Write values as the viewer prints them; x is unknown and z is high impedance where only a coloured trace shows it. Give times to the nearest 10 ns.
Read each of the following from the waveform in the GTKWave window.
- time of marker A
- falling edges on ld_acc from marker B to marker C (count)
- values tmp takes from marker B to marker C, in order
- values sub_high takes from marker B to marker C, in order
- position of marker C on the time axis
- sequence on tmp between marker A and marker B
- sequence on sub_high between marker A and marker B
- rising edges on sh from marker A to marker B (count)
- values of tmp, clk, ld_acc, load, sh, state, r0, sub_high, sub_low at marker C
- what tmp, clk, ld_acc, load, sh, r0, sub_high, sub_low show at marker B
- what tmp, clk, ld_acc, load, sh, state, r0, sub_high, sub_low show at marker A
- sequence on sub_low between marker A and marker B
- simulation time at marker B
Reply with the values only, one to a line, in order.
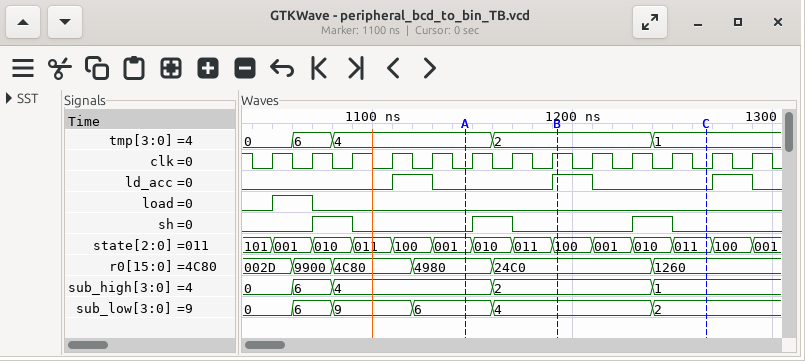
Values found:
1150 ns
1
2, 1
2, 1
1270 ns
4, 2
4, 2
1
tmp=1, clk=0, ld_acc=0, load=0, sh=0, state=011, r0=1260, sub_high=1, sub_low=2
tmp=2, clk=1, ld_acc=1, load=0, sh=0, r0=24C0, sub_high=2, sub_low=4
tmp=4, clk=0, ld_acc=0, load=0, sh=0, state=001, r0=4980, sub_high=4, sub_low=6
6, 4
1190 ns
